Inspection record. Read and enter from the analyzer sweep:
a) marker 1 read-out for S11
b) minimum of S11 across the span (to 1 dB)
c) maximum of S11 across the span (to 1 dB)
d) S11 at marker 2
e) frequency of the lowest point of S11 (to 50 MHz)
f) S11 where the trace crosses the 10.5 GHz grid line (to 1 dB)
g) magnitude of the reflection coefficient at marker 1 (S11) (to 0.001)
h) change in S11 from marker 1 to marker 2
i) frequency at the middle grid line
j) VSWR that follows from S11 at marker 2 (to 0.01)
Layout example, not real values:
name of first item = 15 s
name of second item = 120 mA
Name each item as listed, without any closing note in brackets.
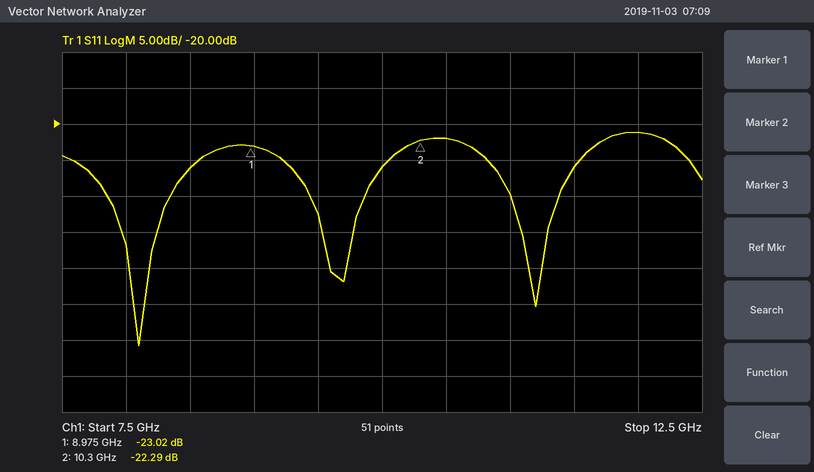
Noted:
marker 1 read-out for S11 = -23.02 dB
minimum of S11 across the span = -51 dB
maximum of S11 across the span = -21 dB
S11 at marker 2 = -22.29 dB
frequency of the lowest point of S11 = 8.10 GHz
S11 where the trace crosses the 10.5 GHz grid line = -22 dB
magnitude of the reflection coefficient at marker 1 (S11) = 0.071
change in S11 from marker 1 to marker 2 = 0.73 dB
frequency at the middle grid line = 10 GHz
VSWR that follows from S11 at marker 2 = 1.17
